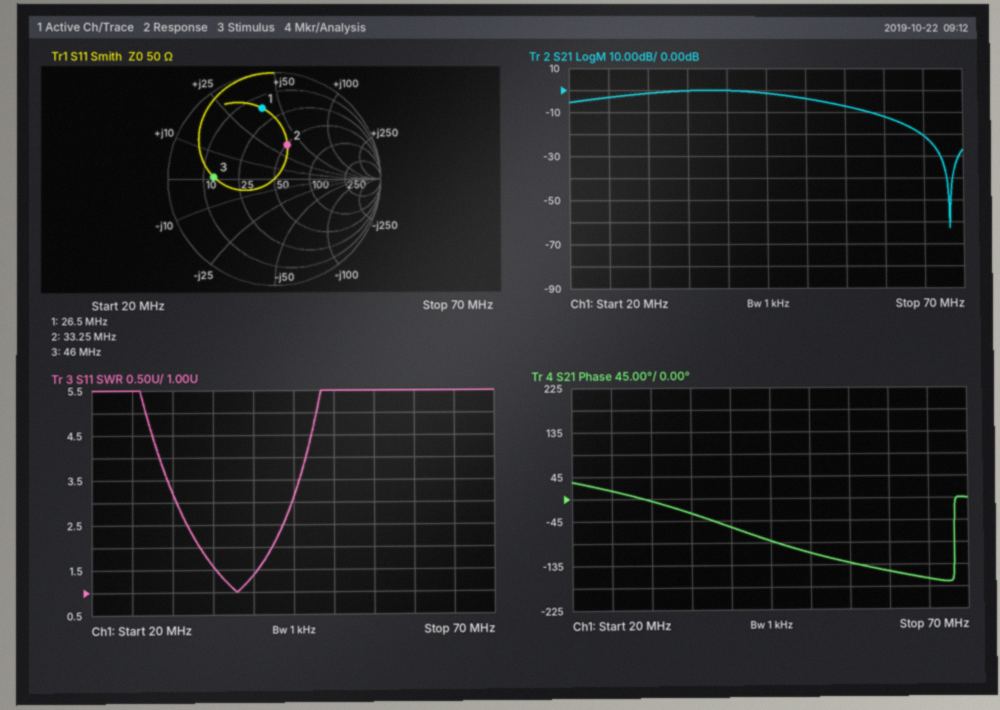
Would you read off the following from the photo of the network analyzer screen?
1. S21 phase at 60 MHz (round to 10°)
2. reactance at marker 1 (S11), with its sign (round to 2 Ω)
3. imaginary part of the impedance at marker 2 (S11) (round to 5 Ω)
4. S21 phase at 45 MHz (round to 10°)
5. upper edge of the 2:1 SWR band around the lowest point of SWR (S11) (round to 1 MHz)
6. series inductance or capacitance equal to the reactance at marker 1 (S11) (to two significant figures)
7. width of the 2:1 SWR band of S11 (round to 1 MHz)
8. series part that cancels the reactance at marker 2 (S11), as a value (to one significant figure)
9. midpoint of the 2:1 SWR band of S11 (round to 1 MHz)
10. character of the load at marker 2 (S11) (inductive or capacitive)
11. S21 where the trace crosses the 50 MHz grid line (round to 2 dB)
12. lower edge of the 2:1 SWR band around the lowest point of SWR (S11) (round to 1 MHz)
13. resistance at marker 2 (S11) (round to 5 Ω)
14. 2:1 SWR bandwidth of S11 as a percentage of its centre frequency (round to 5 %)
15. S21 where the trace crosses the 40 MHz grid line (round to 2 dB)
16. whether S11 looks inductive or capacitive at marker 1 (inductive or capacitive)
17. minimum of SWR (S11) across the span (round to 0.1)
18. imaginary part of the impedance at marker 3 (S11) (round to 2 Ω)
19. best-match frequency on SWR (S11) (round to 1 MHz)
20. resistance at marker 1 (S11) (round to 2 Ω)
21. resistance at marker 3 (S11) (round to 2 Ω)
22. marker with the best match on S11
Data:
-150°
+40 Ω
+35 Ω
-90°
42 MHz
240 nH
9 MHz
100 pF
38 MHz
inductive
-4 dB
33 MHz
50 Ω
25 %
0 dB
inductive
1.0
0 Ω
38 MHz
16 Ω
14 Ω
marker 2
